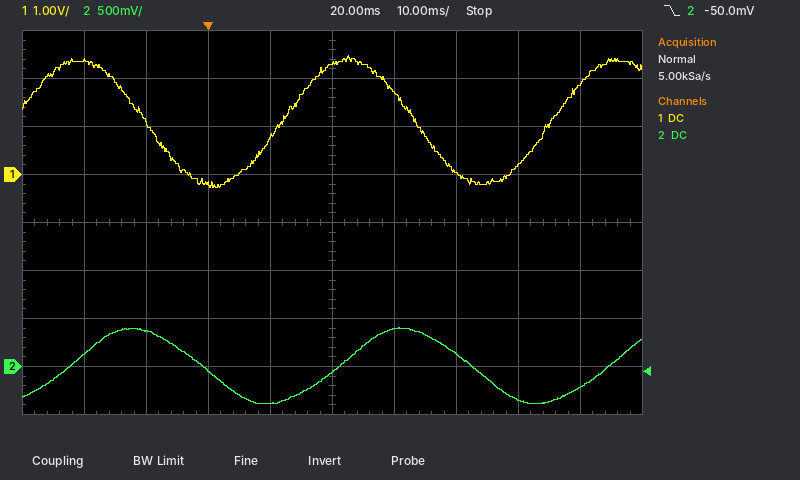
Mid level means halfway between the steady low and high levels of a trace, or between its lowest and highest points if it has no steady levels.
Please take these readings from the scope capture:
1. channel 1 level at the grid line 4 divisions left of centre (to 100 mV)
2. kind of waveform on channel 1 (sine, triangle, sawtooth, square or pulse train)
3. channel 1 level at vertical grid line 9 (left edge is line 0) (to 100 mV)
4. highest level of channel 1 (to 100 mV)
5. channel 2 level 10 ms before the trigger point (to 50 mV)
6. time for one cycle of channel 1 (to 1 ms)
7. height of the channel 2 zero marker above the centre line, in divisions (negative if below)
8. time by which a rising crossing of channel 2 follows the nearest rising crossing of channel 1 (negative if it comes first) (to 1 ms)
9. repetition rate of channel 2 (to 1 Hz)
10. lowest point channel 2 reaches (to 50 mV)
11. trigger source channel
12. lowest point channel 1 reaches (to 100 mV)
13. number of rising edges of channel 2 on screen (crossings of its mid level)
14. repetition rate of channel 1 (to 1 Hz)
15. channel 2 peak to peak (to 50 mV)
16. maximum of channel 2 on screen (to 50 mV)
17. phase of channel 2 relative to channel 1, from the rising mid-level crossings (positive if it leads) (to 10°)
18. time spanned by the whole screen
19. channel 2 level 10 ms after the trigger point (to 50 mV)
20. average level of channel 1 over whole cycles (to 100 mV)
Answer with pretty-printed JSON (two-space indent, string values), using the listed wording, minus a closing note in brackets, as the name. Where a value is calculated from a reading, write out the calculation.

{
  "channel 1 level at the grid line 4 divisions left of centre": "2.4 V",
  "kind of waveform on channel 1": "sine",
  "channel 1 level at vertical grid line 9 (left edge is line 0)": "1.9 V",
  "highest level of channel 1": "2.5 V",
  "channel 2 level 10 ms before the trigger point": "350 mV",
  "time for one cycle of channel 1": "43 ms",
  "height of the channel 2 zero marker above the centre line, in divisions": "-3.0 div",
  "time by which a rising crossing of channel 2 follows the nearest rising crossing of channel 1 (negative if it comes first)": "+9 ms",
  "repetition rate of channel 2": "23 Hz",
  "lowest point channel 2 reaches": "-400 mV",
  "trigger source channel": "channel 2",
  "lowest point channel 1 reaches": "-300 mV",
  "number of rising edges of channel 2 on screen": "3",
  "repetition rate of channel 1": "1 / 43 ms ≈ 23 Hz",
  "channel 2 peak to peak": "400 mV − (-400 mV) = 800 mV",
  "maximum of channel 2 on screen": "400 mV",
  "phase of channel 2 relative to channel 1, from the rising mid-level crossings (positive if it leads)": "−360° × (+9 ms) / 43 ms ≈ -75.3°, so -80° to the nearest 10°",
  "time spanned by the whole screen": "100 ms",
  "channel 2 level 10 ms after the trigger point": "-400 mV",
  "average level of channel 1 over whole cycles": "(2.5 V + (-300 mV)) / 2 ≈ 1.1 V"
}
